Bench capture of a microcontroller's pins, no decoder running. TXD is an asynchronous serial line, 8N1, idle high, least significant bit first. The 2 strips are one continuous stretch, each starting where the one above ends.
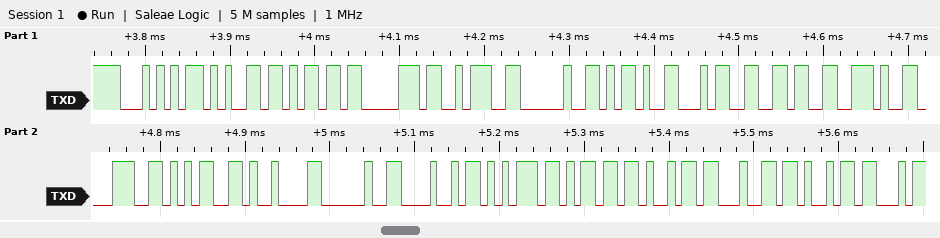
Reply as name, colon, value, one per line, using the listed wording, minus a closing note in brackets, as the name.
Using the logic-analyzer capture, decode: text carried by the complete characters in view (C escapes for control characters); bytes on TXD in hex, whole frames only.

text carried by the complete characters in view: "Temp: -46.85\t Humidi"
bytes on TXD in hex, whole frames only: 54 65 6D 70 3A 20 2D 34 36 2E 38 35 09 20 48 75 6D 69 64 69
